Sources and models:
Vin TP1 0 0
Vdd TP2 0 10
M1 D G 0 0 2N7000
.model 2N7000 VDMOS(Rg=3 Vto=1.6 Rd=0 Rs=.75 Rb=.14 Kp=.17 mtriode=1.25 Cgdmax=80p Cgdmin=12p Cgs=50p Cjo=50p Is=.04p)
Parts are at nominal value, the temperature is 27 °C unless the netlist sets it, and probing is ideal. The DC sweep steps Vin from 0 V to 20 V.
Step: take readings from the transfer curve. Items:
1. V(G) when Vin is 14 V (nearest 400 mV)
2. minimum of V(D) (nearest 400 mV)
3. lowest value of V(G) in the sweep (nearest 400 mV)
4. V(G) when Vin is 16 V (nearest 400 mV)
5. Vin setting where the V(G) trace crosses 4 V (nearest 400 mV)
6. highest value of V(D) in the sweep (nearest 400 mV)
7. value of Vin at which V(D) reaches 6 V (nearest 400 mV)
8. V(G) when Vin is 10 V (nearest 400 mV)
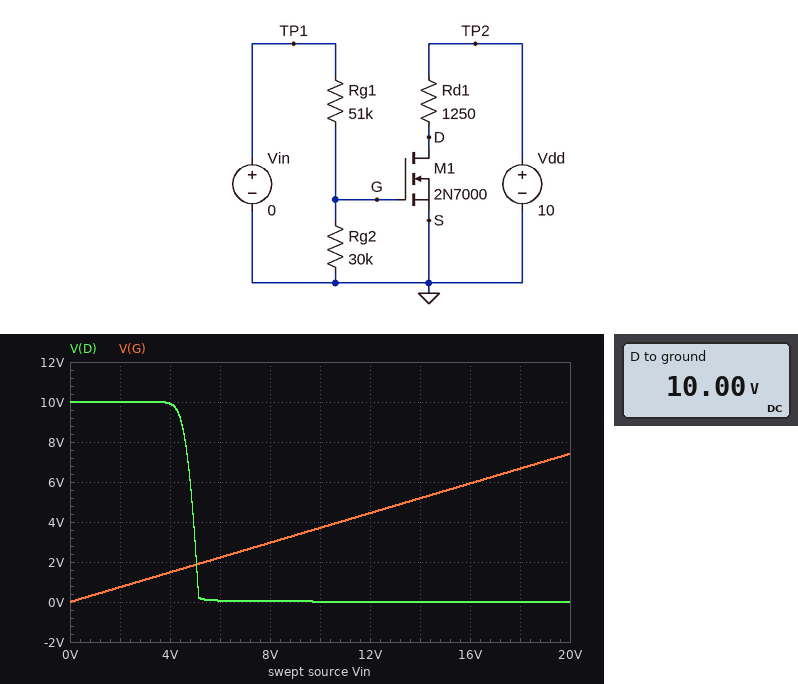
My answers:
5.2 V
0 V
0 V
6.0 V
10.8 V
10.0 V
4.8 V
3.6 V
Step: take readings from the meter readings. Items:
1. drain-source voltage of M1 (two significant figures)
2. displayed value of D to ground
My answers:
10 V
10.00 V
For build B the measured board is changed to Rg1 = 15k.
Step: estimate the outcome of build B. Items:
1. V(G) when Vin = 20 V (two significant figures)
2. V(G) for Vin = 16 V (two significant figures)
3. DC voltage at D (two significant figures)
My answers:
13 V
11 V
10 V
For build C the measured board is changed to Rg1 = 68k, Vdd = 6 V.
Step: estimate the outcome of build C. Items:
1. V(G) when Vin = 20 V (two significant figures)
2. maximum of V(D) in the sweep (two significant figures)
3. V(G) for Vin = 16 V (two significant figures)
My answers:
6.1 V
6.0 V
4.9 V
